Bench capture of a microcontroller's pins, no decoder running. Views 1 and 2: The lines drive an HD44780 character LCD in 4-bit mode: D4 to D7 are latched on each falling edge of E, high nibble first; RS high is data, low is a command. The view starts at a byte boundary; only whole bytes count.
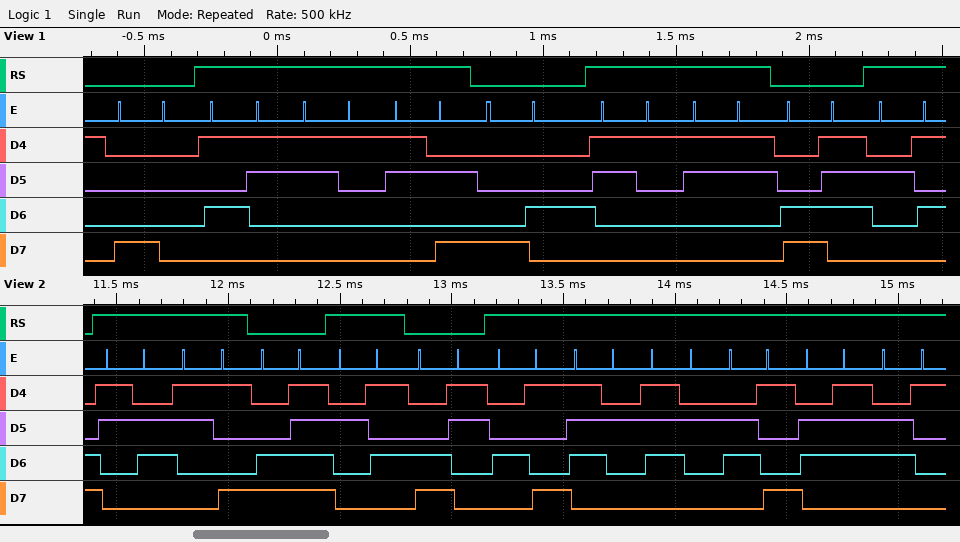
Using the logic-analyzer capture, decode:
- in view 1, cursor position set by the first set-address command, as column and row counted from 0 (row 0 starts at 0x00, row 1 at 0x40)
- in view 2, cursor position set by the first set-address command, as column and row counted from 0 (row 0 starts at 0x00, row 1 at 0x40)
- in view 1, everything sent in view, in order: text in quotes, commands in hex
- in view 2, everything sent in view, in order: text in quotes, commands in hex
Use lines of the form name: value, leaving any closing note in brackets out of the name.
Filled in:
in view 1, cursor position set by the first set-address command, as column and row counted from 0: column 0, row 0
in view 2, cursor position set by the first set-address command, as column and row counted from 0: column 15, row 1
in view 1, everything sent in view, in order: text in quotes, commands in hex: 0x80 "S1:" 0x84 "13" 0xC7 "%"
in view 2, everything sent in view, in order: text in quotes, commands in hex: "69" 0xCF "%" 0xC3 "Irriga"
